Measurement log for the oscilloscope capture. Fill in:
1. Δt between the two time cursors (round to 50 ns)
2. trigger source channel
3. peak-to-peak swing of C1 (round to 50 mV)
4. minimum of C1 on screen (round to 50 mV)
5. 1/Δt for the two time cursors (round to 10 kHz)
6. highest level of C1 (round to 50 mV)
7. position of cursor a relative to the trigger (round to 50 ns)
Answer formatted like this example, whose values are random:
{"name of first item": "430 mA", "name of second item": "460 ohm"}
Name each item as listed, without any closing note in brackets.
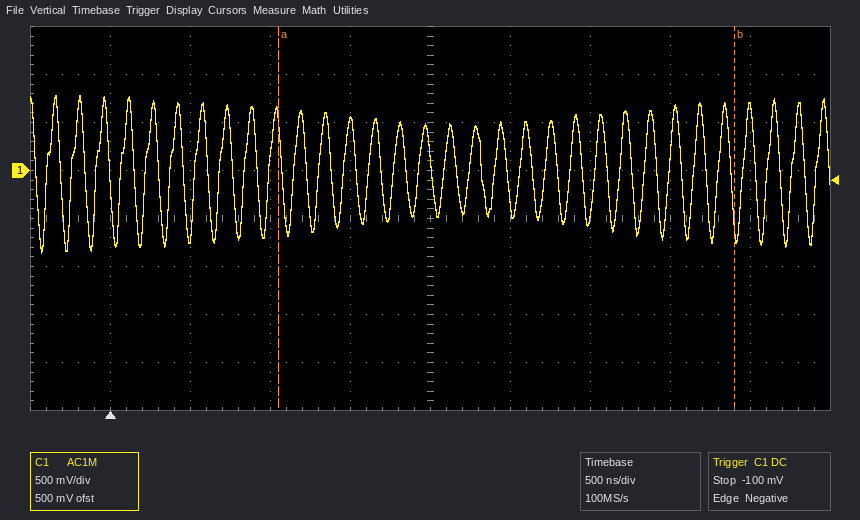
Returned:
{"Δt between the two time cursors": "2.85 µs", "trigger source channel": "C1", "peak-to-peak swing of C1": "1.65 V", "minimum of C1 on screen": "-850 mV", "1/Δt for the two time cursors": "350 kHz", "highest level of C1": "800 mV", "position of cursor a relative to the trigger": "+1.05 µs"}
